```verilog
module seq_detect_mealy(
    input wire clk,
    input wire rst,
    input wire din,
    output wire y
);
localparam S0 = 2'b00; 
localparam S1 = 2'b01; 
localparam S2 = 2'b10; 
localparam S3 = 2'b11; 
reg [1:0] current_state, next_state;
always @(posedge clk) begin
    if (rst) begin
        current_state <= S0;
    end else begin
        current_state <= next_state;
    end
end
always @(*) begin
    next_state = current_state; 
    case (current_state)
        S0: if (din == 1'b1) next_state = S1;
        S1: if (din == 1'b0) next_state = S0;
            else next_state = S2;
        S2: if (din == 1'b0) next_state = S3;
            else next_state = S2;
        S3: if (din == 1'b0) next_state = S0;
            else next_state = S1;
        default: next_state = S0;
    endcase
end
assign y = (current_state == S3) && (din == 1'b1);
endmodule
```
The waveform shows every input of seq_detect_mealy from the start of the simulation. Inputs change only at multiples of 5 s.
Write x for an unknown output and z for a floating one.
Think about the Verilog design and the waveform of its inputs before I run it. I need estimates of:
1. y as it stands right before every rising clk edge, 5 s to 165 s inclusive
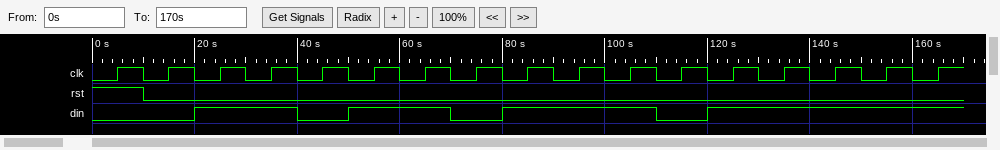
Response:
0 0 0 0 0 1 0 0 1 0 0 0 1 0 0 0 0
